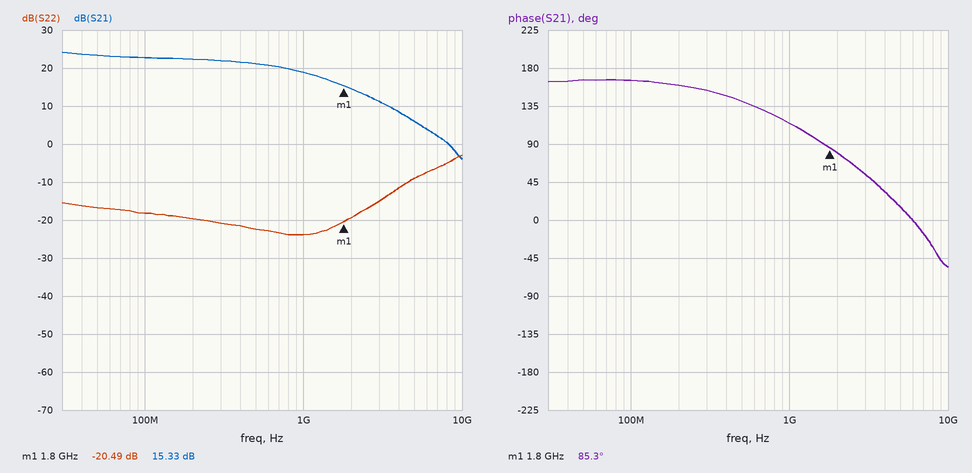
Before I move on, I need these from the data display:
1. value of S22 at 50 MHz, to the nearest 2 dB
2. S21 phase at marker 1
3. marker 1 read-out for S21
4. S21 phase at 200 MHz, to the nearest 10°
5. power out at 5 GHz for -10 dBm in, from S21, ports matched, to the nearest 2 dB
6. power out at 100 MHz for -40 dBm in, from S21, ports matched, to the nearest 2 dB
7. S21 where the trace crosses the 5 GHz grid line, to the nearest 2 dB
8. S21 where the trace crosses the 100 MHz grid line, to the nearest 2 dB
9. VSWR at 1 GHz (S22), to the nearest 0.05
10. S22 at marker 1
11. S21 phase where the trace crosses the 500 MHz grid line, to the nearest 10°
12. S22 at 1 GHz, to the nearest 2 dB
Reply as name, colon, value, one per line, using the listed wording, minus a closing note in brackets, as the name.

value of S22 at 50 MHz, to the nearest 2 dB: -16 dB
S21 phase at marker 1: 85.3°
marker 1 read-out for S21: 15.33 dB
S21 phase at 200 MHz, to the nearest 10°: 160°
power out at 5 GHz for -10 dBm in, from S21, ports matched, to the nearest 2 dB: -4 dBm
power out at 100 MHz for -40 dBm in, from S21, ports matched, to the nearest 2 dB: -18 dBm
S21 where the trace crosses the 5 GHz grid line, to the nearest 2 dB: 6 dB
S21 where the trace crosses the 100 MHz grid line, to the nearest 2 dB: 22 dB
VSWR at 1 GHz (S22), to the nearest 0.05: 1.15
S22 at marker 1: -20.49 dB
S21 phase where the trace crosses the 500 MHz grid line, to the nearest 10°: 140°
S22 at 1 GHz, to the nearest 2 dB: -24 dB
